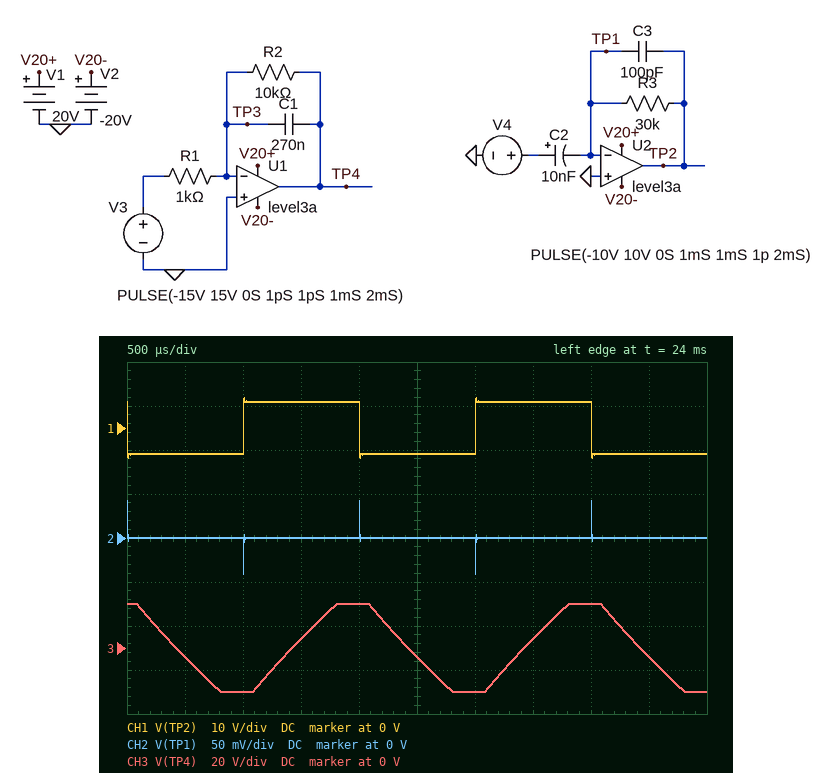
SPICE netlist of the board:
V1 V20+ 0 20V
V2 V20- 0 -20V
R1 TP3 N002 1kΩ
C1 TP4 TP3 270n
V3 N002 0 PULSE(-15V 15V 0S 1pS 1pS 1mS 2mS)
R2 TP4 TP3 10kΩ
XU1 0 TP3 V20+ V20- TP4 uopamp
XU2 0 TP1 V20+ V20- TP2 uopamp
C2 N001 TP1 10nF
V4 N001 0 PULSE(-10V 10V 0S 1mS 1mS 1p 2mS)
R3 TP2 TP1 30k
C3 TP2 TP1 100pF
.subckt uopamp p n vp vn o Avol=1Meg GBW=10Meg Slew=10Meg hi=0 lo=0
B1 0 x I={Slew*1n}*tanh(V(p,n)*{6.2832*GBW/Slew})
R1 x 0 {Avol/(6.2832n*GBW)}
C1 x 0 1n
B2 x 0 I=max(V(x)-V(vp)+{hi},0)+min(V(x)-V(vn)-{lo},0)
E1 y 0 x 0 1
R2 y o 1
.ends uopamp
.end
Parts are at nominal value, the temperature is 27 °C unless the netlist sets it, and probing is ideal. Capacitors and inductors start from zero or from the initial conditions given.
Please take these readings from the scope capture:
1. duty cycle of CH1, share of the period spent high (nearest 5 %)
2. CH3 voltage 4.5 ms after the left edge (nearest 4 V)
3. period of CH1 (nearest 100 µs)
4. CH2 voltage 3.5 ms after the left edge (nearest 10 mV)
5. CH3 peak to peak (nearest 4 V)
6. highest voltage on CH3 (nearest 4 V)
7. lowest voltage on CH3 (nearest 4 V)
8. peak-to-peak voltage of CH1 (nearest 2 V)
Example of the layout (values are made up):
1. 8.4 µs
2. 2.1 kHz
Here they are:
1. 50 %
2. -4 V
3. 2.0 ms
4. 0 V
5. 40 V
6. 20 V
7. -20 V
8. 14 V
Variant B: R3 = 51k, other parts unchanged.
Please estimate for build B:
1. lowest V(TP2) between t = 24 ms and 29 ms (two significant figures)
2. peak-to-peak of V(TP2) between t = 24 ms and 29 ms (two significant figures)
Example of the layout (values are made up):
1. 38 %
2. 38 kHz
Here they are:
1. -10 V
2. 21 V
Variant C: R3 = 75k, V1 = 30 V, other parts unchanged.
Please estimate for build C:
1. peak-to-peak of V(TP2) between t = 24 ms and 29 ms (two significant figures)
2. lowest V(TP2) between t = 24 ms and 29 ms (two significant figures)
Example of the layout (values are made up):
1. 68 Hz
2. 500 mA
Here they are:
1. 30 V
2. -15 V
